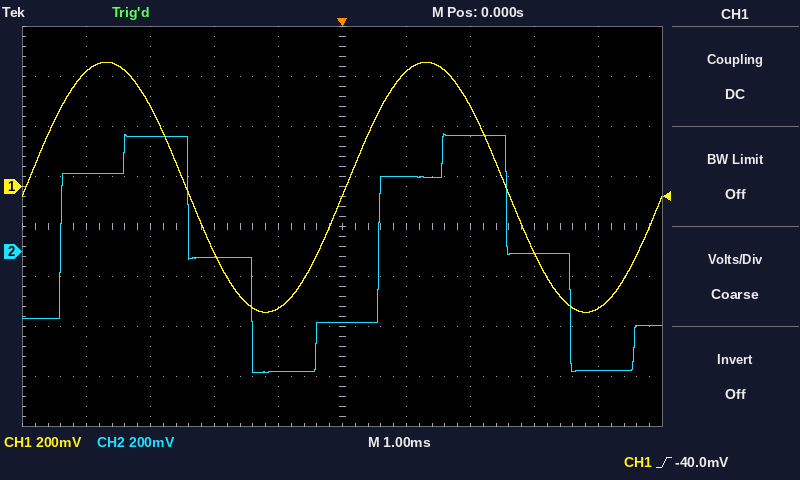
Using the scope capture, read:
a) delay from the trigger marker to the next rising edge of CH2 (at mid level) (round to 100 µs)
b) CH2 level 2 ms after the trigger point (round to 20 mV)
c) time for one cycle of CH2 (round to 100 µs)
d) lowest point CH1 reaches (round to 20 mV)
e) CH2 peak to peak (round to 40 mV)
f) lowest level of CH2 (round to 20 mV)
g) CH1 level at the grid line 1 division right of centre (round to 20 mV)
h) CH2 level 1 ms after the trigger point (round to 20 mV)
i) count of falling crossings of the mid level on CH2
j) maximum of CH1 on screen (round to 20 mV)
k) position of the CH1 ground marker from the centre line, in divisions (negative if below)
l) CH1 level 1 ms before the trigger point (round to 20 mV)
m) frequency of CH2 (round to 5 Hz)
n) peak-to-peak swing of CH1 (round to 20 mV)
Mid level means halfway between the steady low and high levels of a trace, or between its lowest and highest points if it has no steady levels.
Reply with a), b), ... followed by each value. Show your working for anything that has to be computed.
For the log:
a) 600 µs
b) 460 mV
c) 5.0 ms
d) -500 mV
e) 960 mV
f) -480 mV
g) 460 mV
h) 300 mV
i) 2
j) 500 mV
k) +0.8 div
l) -480 mV
m) 1 / 5.0 ms ≈ 200 Hz
n) 500 mV − (-500 mV) = 1.00 V
